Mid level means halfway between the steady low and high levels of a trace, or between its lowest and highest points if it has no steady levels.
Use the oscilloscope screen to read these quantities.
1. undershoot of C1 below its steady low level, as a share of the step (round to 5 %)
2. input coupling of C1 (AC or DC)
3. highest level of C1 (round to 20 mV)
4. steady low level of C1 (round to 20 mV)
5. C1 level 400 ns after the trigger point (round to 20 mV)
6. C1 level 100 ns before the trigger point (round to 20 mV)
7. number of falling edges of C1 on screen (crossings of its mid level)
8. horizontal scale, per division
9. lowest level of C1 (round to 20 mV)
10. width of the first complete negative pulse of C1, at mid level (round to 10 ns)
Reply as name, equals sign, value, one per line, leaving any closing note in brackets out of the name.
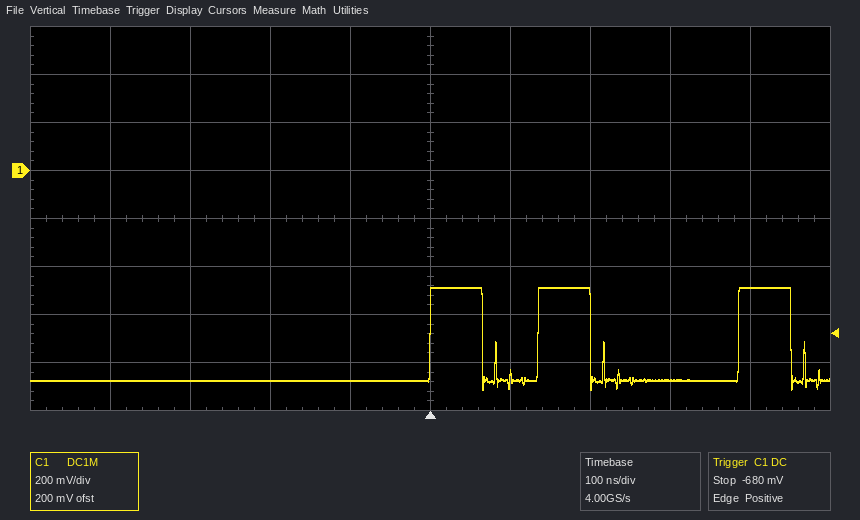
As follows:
undershoot of C1 below its steady low level, as a share of the step = 10 %
input coupling of C1 = DC
highest level of C1 = -480 mV
steady low level of C1 = -880 mV
C1 level 400 ns after the trigger point = -480 mV
C1 level 100 ns before the trigger point = -880 mV
number of falling edges of C1 on screen = 3
horizontal scale, per division = 100 ns
lowest level of C1 = -920 mV
width of the first complete negative pulse of C1, at mid level = 70 ns
